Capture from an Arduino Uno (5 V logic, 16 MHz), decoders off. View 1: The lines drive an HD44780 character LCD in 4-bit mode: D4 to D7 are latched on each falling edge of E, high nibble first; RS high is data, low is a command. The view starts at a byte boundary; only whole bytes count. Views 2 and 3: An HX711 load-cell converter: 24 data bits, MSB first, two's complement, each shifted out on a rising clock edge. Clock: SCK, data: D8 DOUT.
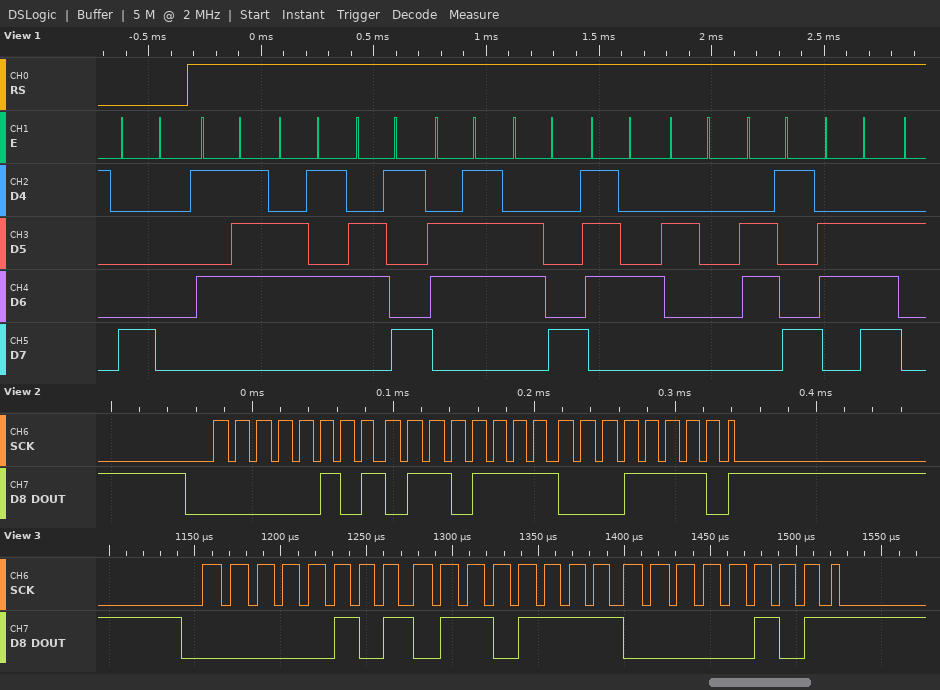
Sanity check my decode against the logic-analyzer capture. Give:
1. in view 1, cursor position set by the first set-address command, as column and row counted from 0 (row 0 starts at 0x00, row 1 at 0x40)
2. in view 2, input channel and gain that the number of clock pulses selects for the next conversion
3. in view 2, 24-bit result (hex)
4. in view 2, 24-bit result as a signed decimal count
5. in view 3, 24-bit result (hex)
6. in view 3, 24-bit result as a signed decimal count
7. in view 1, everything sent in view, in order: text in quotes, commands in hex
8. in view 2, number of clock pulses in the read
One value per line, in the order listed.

column 0, row 0
channel A, gain 128
0x056F1E
356126
0x056F05
356101
0x80 "Weight in"
25
